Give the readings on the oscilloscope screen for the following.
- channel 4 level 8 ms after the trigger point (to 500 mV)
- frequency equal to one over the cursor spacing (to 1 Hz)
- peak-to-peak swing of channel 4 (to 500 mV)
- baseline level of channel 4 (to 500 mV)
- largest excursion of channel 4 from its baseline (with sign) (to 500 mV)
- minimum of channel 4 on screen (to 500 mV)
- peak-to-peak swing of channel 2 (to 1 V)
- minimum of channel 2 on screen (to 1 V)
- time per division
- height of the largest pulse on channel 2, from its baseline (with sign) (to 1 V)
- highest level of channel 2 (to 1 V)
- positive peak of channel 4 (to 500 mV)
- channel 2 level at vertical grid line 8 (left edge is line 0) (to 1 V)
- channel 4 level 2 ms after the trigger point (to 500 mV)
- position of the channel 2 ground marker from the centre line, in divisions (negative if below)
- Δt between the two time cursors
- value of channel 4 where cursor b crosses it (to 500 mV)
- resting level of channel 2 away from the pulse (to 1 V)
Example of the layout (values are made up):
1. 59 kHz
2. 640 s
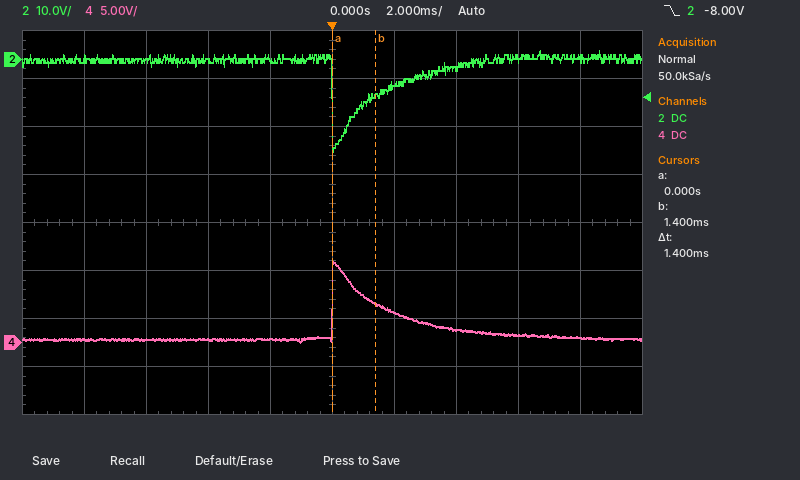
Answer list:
1. 500 mV
2. 714 Hz
3. 8.5 V
4. 500 mV
5. +8.0 V
6. 0.0 V
7. 21 V
8. -19 V
9. 2 ms
10. -19 V
11. 2 V
12. 8.5 V
13. 0 V
14. 3.0 V
15. +3.4 div
16. 1.4 ms
17. 4.0 V
18. 0 V
